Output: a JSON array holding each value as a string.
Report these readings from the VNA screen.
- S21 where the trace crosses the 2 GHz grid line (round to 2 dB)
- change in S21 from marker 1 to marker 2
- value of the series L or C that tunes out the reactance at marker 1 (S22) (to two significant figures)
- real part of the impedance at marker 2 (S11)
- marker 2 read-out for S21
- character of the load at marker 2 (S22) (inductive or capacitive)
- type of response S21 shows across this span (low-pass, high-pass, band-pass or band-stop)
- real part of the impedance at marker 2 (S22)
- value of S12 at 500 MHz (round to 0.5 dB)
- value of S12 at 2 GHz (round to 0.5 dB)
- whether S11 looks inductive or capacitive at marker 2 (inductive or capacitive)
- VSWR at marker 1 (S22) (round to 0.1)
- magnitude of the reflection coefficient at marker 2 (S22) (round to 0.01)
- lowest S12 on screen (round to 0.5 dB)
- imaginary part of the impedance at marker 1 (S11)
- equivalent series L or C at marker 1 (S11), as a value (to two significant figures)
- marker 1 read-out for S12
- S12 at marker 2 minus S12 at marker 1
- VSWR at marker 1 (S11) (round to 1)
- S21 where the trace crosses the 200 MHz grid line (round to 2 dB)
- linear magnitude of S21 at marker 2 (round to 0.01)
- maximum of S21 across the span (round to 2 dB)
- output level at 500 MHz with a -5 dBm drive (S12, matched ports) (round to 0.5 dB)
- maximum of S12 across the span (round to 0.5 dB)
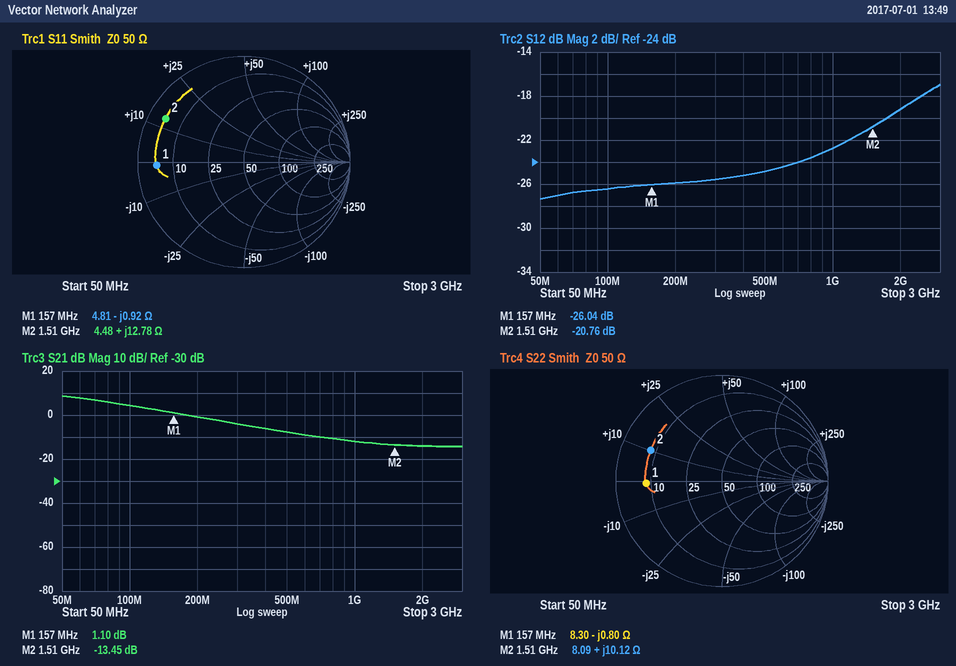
["-14 dB", "-14.55 dB", "810 pH", "4.48 Ω", "-13.45 dB", "inductive", "low-pass", "8.09 Ω", "-25.0 dB", "-19.0 dB", "inductive", "6.0", "0.73", "-27.5 dB", "-0.92 Ω", "1.1 nF", "-26.04 dB", "5.28 dB", "10", "0 dB", "0.21", "8 dB", "-30.0 dBm", "-17.0 dB"]
